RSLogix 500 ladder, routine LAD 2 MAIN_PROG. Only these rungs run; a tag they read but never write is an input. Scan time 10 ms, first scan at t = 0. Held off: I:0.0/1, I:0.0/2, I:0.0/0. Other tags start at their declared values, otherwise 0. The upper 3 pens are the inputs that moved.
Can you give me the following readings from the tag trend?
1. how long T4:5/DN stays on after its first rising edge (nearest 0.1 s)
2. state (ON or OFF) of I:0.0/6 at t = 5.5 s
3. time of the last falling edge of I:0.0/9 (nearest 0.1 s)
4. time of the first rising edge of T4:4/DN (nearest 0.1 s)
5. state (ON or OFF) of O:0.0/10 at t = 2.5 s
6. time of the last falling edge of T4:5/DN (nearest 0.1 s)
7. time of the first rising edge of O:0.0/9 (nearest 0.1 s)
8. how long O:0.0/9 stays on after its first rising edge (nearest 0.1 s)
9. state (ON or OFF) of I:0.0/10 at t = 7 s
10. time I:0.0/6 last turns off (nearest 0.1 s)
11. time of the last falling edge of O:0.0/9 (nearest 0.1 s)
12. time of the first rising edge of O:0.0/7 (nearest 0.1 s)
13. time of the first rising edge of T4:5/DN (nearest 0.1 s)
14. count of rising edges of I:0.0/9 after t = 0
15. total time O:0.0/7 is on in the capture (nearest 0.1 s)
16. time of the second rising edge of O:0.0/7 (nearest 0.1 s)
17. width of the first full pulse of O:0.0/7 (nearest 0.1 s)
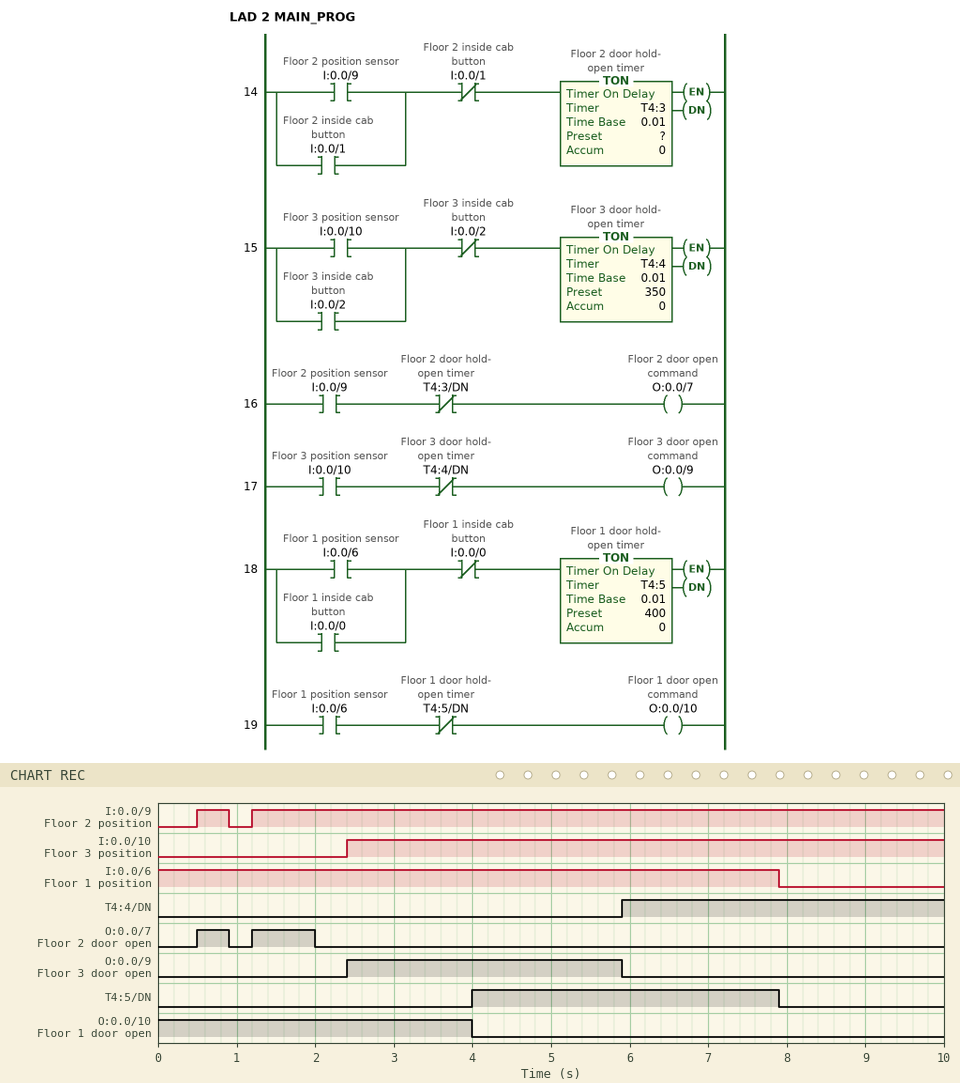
3.9 s
ON
0.9 s
5.9 s
ON
7.9 s
2.4 s
3.5 s
ON
7.9 s
5.9 s
0.5 s
4.0 s
2
1.2 s
1.2 s
0.4 s
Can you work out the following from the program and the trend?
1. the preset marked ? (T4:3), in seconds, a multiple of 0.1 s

0.8 s
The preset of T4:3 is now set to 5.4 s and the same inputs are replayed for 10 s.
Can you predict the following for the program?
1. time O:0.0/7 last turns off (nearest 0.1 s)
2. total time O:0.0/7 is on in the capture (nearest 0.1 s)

6.6 s
5.8 s
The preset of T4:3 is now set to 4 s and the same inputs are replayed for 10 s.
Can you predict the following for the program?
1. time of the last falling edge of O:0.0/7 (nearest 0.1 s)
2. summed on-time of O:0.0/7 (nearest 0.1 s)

5.2 s
4.4 s
